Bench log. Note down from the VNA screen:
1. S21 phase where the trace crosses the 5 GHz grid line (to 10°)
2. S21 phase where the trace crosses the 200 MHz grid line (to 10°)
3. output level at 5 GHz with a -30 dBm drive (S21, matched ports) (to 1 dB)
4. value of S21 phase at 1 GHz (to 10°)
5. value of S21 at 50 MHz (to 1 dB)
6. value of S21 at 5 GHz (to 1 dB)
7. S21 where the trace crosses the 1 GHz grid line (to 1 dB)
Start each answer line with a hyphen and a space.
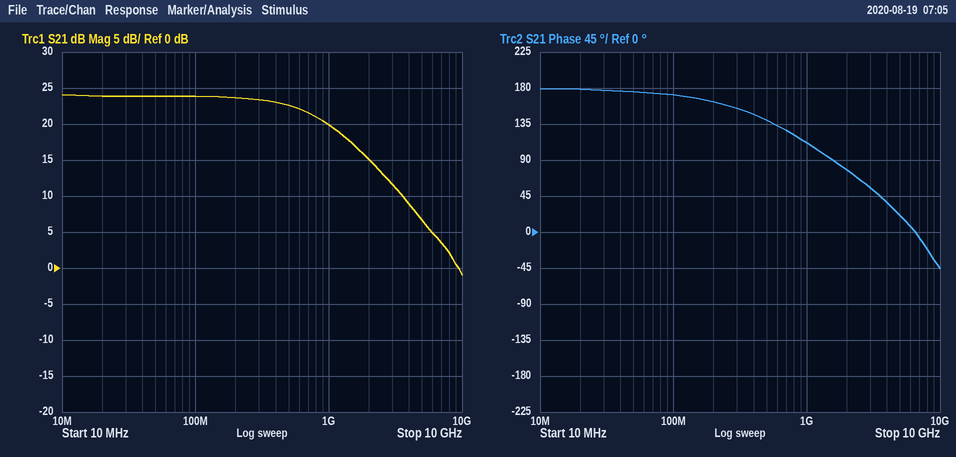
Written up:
- 20°
- 160°
- -23 dBm
- 110°
- 24 dB
- 7 dB
- 20 dB
